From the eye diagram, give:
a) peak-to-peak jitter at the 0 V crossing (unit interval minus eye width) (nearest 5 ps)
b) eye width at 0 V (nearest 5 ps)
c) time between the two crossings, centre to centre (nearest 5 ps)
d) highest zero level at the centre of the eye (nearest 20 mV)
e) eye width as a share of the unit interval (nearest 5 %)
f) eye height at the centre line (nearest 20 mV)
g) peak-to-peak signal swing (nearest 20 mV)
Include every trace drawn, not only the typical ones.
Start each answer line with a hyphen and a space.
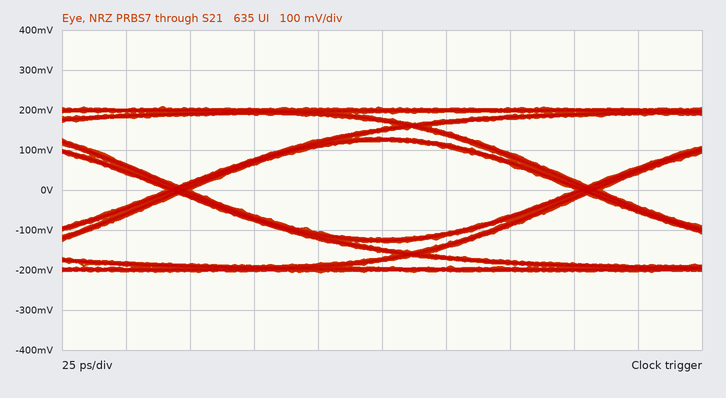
- 10 ps
- 150 ps
- 160 ps
- -120 mV
- 95 %
- 240 mV
- 420 mV
